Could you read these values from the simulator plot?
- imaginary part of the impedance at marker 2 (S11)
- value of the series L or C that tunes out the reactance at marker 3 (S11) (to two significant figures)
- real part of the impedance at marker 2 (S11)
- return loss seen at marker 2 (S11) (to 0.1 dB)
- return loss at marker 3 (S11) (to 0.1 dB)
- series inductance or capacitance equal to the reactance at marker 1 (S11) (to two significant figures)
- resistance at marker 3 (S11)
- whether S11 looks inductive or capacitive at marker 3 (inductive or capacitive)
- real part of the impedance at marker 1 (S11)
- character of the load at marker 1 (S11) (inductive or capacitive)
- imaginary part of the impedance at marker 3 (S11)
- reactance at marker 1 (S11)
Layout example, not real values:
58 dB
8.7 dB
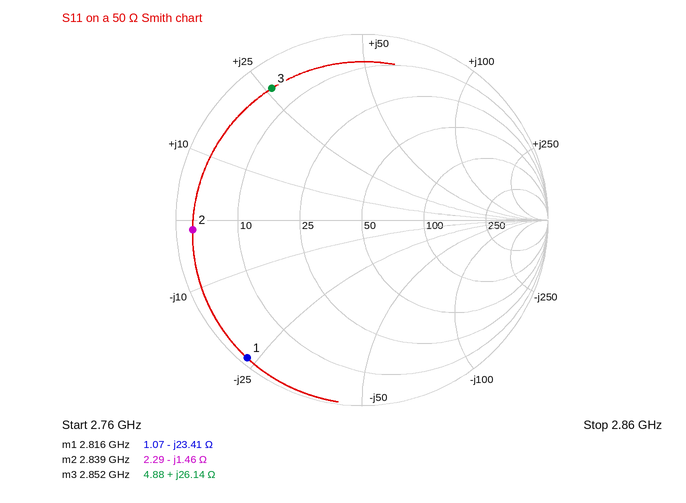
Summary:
-1.46 Ω
2.1 pF
2.29 Ω
0.8 dB
1.3 dB
2.4 pF
4.88 Ω
inductive
1.07 Ω
capacitive
+26.14 Ω
-23.41 Ω
